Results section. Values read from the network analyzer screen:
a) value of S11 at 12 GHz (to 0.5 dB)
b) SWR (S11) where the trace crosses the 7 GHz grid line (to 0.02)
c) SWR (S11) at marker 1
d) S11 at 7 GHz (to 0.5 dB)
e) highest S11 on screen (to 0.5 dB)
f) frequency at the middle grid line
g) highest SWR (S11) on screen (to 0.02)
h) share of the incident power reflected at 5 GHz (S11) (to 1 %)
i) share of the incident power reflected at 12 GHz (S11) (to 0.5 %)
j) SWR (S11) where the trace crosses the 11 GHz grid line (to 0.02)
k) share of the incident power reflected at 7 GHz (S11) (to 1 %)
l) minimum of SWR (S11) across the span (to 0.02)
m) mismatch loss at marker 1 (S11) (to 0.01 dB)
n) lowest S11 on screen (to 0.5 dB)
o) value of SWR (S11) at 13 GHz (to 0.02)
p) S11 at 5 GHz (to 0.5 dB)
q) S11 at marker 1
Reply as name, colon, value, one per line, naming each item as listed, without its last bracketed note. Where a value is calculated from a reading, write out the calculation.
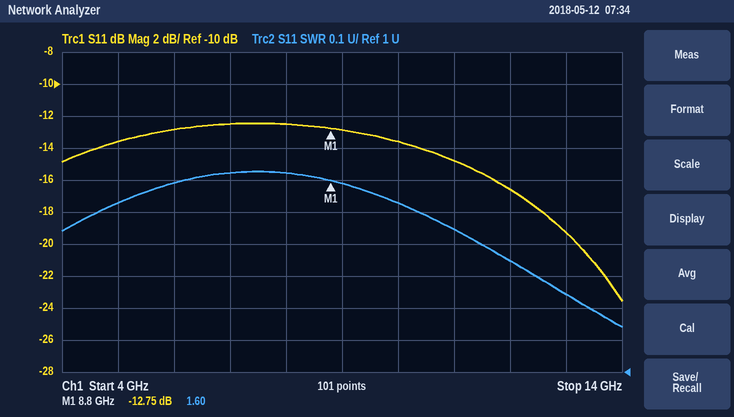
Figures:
value of S11 at 12 GHz: -16.5 dB
SWR (S11) where the trace crosses the 7 GHz grid line: 1.62
SWR (S11) at marker 1: 1.60
S11 at 7 GHz: -12.5 dB
highest S11 on screen: -12.5 dB
frequency at the middle grid line: 9 GHz
highest SWR (S11) on screen: 1.62
share of the incident power reflected at 5 GHz (S11): 10^(-13.5/10) ≈ 4 %
share of the incident power reflected at 12 GHz (S11): 10^(-16.5/10) ≈ 2.24 %, so 2.0 % to the nearest 0.5 %
SWR (S11) where the trace crosses the 11 GHz grid line: 1.44
share of the incident power reflected at 7 GHz (S11): 10^(-12.5/10) ≈ 6 %
minimum of SWR (S11) across the span: 1.14
mismatch loss at marker 1 (S11): −10 log10(1 − 10^(-12.75/10)) ≈ 0.24 dB
lowest S11 on screen: -23.5 dB
value of SWR (S11) at 13 GHz: 1.24
S11 at 5 GHz: -13.5 dB
S11 at marker 1: -12.75 dB
